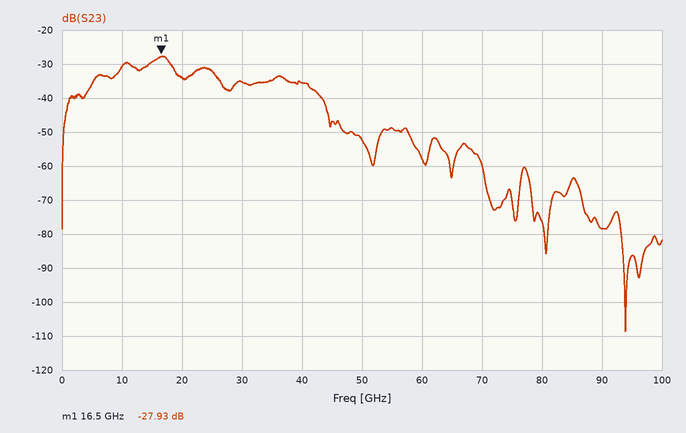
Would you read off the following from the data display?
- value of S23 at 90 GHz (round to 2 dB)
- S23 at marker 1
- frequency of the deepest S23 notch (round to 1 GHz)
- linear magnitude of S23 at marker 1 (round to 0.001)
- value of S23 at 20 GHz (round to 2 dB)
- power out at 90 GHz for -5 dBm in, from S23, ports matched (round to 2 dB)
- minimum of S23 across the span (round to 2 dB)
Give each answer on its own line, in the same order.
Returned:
-78 dB
-27.93 dB
94 GHz
0.040
-34 dB
-84 dBm
-108 dB
